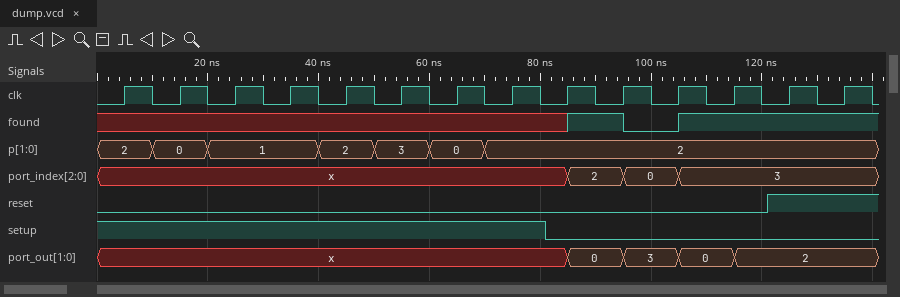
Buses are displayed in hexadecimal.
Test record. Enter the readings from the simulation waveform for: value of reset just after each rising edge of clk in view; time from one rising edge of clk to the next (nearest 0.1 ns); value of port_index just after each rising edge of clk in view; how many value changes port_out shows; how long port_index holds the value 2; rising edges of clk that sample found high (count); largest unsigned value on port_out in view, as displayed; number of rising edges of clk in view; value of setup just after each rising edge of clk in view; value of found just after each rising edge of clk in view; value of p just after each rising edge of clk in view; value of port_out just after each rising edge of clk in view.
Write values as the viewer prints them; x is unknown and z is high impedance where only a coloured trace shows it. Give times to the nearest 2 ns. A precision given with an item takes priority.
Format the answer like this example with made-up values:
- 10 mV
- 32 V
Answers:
- 0 0 0 0 0 0 0 0 0 0 0 0 1 1
- 10 ns
- x, x, x, x, x, x, x, x, 2, 0, 3, 3, 3, 3
- 4
- 10 ns
- 4
- 3
- 14
- 1 1 1 1 1 1 1 1 0 0 0 0 0 0
- x x x x x x x x 1 0 1 1 1 1
- 2, 0, 1, 1, 2, 3, 0, 2, 2, 2, 2, 2, 2, 2
- x, x, x, x, x, x, x, x, 0, 3, 0, 2, 2, 2
